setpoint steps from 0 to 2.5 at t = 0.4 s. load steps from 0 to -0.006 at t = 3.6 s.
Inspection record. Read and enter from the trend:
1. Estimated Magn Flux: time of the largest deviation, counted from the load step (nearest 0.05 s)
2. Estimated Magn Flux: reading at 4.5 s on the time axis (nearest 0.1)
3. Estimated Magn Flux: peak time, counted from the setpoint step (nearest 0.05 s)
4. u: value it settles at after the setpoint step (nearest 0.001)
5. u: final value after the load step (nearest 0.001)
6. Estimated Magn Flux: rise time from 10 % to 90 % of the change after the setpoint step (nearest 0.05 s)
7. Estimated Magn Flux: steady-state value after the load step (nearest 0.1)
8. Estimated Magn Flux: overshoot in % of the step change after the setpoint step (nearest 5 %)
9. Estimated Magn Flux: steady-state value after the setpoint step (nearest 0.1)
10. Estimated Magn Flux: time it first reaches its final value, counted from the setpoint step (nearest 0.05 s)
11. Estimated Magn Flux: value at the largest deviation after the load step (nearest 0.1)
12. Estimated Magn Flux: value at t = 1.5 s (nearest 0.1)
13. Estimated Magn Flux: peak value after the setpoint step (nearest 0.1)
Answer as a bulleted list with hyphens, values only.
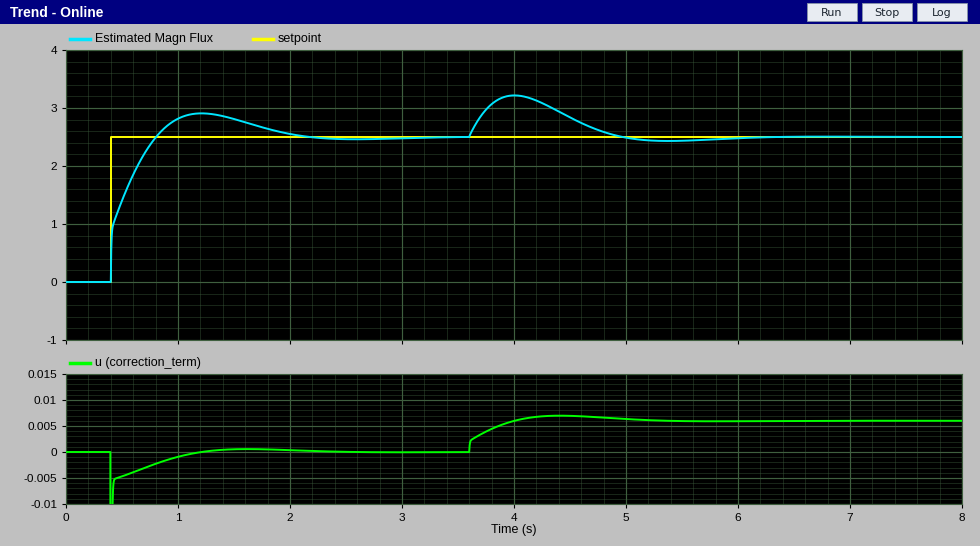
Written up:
- 0.40 s
- 2.8
- 0.80 s
- 0.000
- 0.006
- 0.30 s
- 2.5
- 15 %
- 2.5
- 0.40 s
- 3.2
- 2.8
- 2.9
